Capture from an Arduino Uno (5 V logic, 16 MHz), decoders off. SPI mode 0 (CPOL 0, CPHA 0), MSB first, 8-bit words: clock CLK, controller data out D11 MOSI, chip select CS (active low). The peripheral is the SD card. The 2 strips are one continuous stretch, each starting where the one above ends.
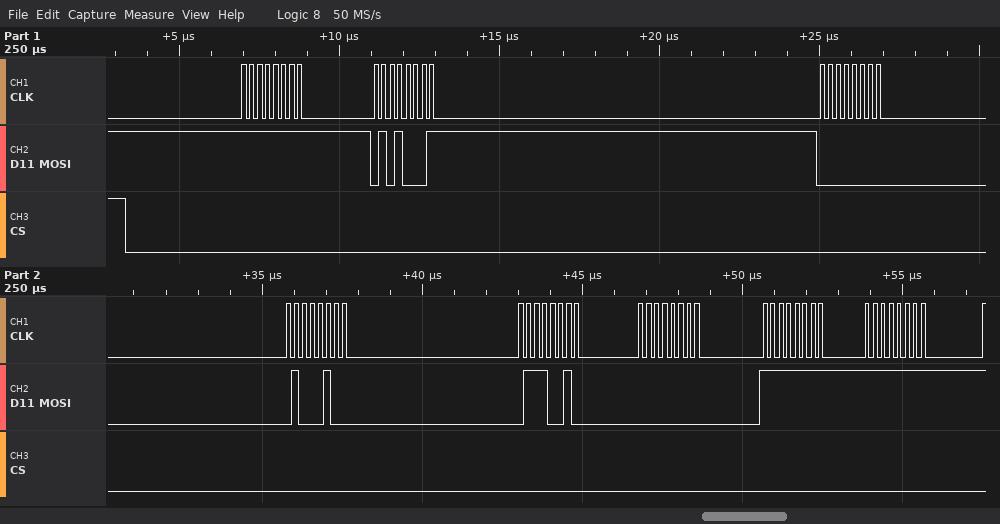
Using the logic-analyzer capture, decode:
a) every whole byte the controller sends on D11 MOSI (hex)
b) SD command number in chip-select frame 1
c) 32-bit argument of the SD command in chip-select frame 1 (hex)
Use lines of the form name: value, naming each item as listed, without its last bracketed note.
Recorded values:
every whole byte the controller sends on D11 MOSI: FF 51 00 44 72 00 FF FF
SD command number in chip-select frame 1: CMD17
32-bit argument of the SD command in chip-select frame 1: 0x00447200
